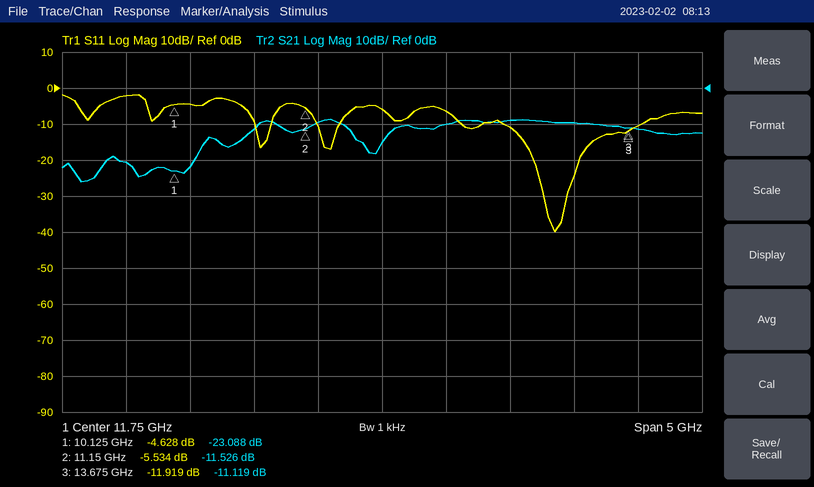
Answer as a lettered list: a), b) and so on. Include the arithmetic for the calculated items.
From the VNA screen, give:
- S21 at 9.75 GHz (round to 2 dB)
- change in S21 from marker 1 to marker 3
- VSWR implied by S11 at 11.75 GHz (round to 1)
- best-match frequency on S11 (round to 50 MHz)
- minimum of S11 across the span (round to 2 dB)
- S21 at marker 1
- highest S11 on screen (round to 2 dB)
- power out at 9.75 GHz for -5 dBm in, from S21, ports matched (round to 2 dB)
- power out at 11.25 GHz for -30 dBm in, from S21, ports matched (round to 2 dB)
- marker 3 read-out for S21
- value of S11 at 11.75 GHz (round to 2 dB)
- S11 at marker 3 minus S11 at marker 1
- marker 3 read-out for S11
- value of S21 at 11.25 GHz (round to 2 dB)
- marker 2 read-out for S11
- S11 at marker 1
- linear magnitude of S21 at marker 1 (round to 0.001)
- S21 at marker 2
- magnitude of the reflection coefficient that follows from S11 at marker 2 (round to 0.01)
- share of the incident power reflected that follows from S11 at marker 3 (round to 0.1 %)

a) -20 dB
b) -11.119 − (-23.088) = 11.969 dB
c) |Γ| = 10^(-6/20) = 0.5012; VSWR = (1 + 0.5012)/(1 − 0.5012) ≈ 3
d) 13.10 GHz
e) -40 dB
f) -23.088 dB
g) -2 dB
h) -5 dBm + (-20 dB) = -26 dBm
i) -30 dBm + (-10 dB) = -40 dBm
j) -11.119 dB
k) -6 dB
l) -11.919 − (-4.628) = -7.291 dB
m) -11.919 dB
n) -10 dB
o) -5.534 dB
p) -4.628 dB
q) 10^(-23.088/20) ≈ 0.070
r) -11.526 dB
s) 10^(-5.534/20) ≈ 0.53
t) 10^(-11.919/10) ≈ 6.4 %
